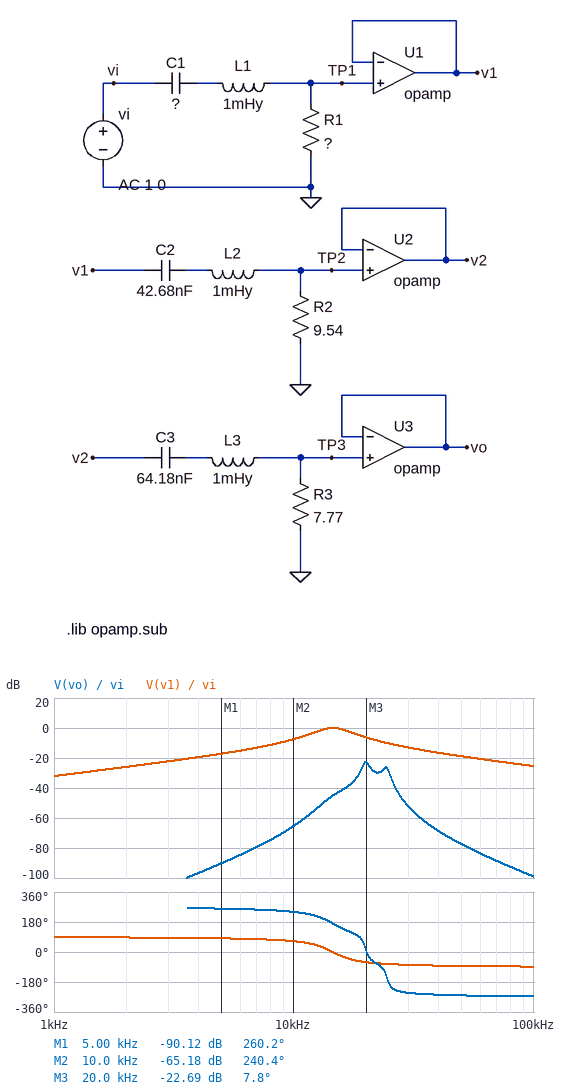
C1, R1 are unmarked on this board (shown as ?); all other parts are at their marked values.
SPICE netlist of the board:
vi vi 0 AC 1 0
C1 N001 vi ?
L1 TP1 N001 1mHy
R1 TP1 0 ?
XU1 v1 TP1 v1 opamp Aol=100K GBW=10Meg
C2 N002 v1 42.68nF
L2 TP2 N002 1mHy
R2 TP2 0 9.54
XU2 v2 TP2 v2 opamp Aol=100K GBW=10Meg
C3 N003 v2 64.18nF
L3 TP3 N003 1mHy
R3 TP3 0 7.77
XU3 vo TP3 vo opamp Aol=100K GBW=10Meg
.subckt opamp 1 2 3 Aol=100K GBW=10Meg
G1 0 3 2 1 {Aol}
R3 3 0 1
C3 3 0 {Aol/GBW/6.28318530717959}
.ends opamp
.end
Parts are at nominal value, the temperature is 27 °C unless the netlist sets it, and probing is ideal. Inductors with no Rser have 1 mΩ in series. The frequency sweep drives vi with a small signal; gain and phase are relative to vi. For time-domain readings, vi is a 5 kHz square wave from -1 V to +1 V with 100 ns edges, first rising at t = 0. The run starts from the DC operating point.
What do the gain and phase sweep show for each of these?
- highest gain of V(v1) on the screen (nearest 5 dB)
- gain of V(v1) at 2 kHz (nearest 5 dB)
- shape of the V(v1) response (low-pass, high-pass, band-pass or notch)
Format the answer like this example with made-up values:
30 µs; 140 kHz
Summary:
0 dB; -25 dB; band-pass
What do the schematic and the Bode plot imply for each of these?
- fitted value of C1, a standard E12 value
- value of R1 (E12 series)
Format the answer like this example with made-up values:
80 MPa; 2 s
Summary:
120 nF; 33 Ω
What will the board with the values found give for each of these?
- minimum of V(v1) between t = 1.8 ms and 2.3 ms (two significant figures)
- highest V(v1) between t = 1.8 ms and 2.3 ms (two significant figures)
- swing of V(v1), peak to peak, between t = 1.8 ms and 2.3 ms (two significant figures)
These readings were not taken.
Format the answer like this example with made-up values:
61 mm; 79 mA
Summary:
-660 mV; 660 mV; 1.3 V
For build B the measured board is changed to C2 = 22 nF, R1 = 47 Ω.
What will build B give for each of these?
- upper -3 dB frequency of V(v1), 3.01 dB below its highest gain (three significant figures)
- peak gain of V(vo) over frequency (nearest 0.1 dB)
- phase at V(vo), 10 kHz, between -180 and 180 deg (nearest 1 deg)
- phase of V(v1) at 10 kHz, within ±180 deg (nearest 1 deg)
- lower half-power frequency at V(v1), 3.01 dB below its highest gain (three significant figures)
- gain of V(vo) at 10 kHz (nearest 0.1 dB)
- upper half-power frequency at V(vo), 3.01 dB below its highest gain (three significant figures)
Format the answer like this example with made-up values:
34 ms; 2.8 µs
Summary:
18.7 kHz; -32.0 dB; -127 deg; 56 deg; 11.3 kHz; -69.4 dB; 20.5 kHz
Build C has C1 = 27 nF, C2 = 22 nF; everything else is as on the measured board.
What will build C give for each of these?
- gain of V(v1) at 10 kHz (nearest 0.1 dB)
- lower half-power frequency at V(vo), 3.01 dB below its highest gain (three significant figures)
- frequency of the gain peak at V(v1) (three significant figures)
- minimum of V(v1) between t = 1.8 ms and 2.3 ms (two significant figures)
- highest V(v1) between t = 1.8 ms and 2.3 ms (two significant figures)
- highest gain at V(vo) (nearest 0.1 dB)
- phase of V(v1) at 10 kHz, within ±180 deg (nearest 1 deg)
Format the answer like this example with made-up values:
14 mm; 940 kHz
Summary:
-24.1 dB; 32.8 kHz; 30.6 kHz; -250 mV; 250 mV; -28.9 dB; 86 deg
